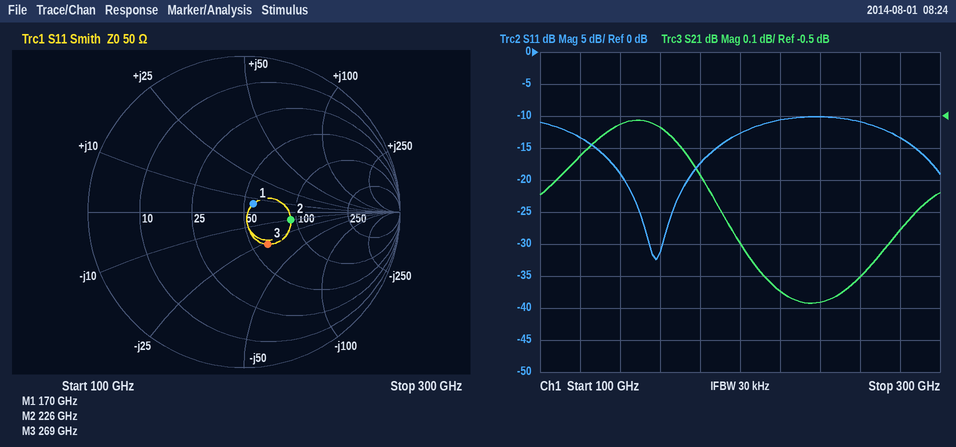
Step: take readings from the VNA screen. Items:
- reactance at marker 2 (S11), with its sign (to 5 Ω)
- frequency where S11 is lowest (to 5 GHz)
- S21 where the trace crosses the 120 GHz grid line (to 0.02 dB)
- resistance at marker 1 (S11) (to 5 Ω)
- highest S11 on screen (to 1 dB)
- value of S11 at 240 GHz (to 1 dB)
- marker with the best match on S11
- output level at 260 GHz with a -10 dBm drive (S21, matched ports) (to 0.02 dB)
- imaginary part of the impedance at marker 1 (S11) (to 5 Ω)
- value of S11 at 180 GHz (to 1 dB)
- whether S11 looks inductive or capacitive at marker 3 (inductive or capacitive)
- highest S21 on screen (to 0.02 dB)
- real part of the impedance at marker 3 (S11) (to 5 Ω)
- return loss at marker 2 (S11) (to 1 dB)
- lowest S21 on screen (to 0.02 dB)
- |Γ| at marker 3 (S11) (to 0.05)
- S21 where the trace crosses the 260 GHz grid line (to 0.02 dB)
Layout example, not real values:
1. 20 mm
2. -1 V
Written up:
1. -10 Ω
2. 160 GHz
3. -0.62 dB
4. 55 Ω
5. -10 dB
6. -10 dB
7. marker 1
8. -11.00 dBm
9. +5 Ω
10. -17 dB
11. capacitive
12. -0.52 dB
13. 60 Ω
14. 10 dB
15. -1.08 dB
16. 0.25
17. -1.00 dB
